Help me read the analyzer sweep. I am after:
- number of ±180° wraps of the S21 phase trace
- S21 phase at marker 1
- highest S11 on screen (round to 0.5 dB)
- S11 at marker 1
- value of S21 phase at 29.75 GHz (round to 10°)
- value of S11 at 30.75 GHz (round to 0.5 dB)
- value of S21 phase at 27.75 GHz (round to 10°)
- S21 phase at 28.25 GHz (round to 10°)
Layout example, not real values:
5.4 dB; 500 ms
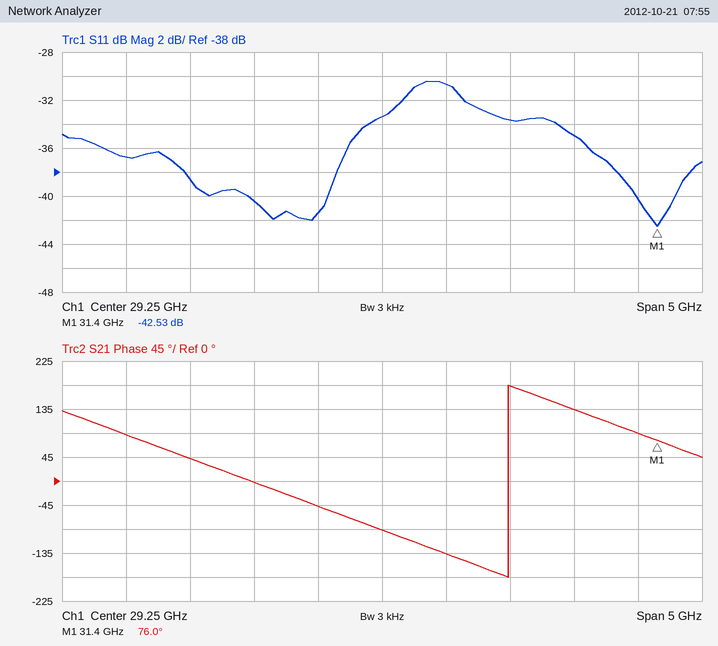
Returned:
1; 76.0°; -30.5 dB; -42.53 dB; -140°; -35.0 dB; 40°; 0°
